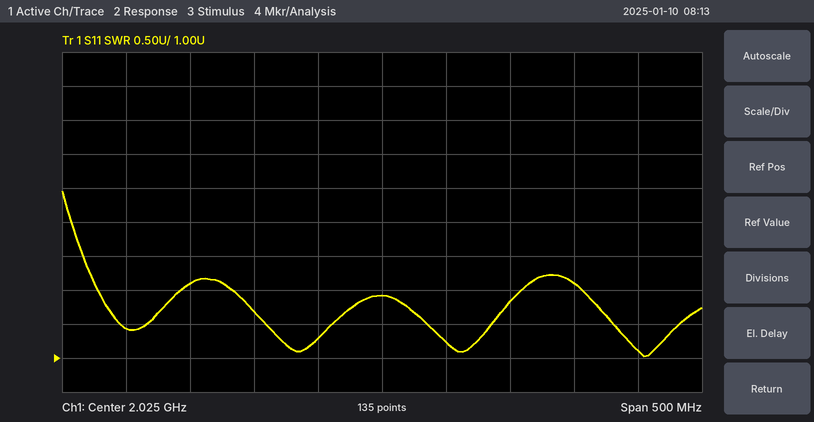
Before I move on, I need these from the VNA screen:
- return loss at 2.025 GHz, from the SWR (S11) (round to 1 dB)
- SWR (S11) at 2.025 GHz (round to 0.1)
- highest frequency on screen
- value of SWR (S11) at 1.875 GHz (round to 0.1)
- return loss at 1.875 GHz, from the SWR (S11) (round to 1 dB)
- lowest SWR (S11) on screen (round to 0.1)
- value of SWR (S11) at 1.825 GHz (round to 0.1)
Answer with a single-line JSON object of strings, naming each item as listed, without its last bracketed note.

{"return loss at 2.025 GHz, from the SWR (S11)": "10 dB", "SWR (S11) at 2.025 GHz": "1.9", "highest frequency on screen": "2.275 GHz", "value of SWR (S11) at 1.875 GHz": "2.1", "return loss at 1.875 GHz, from the SWR (S11)": "9 dB", "lowest SWR (S11) on screen": "1.0", "value of SWR (S11) at 1.825 GHz": "1.4"}
